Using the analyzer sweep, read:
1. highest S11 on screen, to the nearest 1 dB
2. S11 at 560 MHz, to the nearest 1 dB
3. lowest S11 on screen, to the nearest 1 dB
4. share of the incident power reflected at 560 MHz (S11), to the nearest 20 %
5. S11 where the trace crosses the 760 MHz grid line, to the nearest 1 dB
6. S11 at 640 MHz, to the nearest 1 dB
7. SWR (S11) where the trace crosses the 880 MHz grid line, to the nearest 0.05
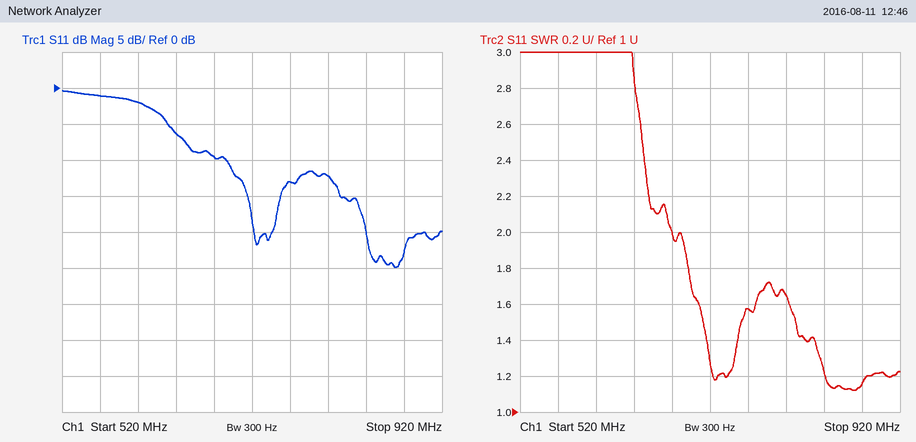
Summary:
0 dB
-1 dB
-25 dB
80 %
-13 dB
-6 dB
1.15
